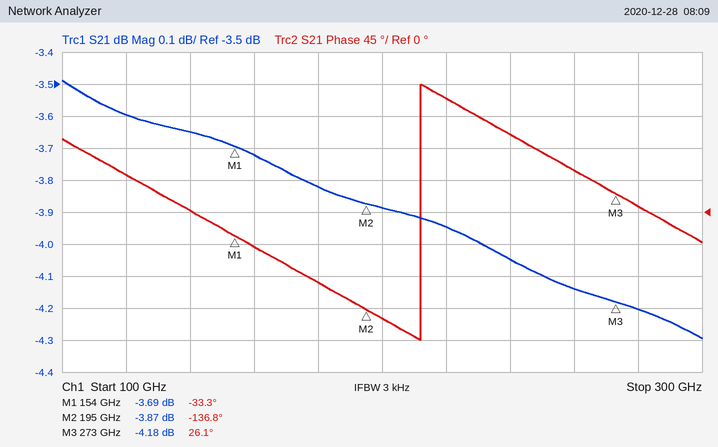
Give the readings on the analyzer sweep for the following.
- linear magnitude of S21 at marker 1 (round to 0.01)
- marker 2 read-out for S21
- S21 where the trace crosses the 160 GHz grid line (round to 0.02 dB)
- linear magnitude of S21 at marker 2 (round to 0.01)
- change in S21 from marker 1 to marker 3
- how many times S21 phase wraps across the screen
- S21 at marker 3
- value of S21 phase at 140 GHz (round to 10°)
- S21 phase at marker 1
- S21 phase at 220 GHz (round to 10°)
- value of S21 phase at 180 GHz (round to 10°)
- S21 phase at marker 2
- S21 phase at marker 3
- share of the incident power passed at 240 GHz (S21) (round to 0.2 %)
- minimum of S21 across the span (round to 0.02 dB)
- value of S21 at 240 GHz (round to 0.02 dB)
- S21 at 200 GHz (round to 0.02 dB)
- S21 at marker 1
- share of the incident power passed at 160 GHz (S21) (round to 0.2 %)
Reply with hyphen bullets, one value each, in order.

- 0.65
- -3.87 dB
- -3.72 dB
- 0.64
- -0.49 dB
- 1
- -4.18 dB
- 0°
- -33.3°
- 160°
- -100°
- -136.8°
- 26.1°
- 39.4 %
- -4.30 dB
- -4.04 dB
- -3.88 dB
- -3.69 dB
- 42.4 %
